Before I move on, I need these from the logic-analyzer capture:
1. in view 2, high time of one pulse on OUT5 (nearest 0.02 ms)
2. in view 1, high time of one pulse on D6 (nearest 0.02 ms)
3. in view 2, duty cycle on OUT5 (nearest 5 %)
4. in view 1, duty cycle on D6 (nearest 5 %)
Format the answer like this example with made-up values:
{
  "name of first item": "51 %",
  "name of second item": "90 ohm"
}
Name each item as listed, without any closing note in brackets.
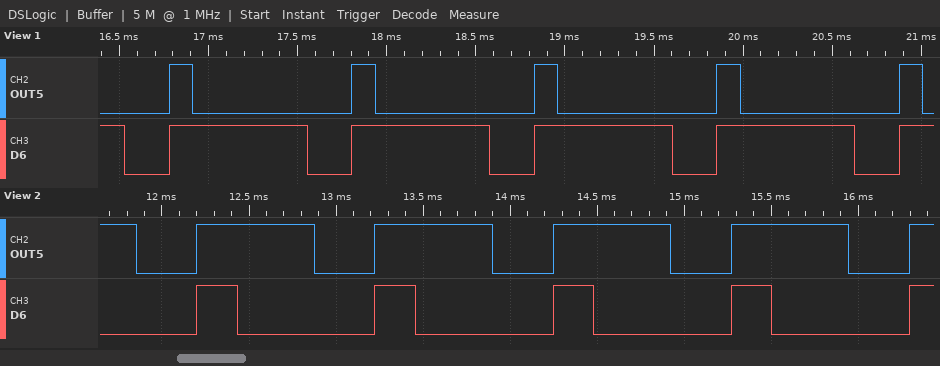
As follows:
{
  "in view 2, high time of one pulse on OUT5": "0.68 ms",
  "in view 1, high time of one pulse on D6": "0.78 ms",
  "in view 2, duty cycle on OUT5": "65 %",
  "in view 1, duty cycle on D6": "75 %"
}
